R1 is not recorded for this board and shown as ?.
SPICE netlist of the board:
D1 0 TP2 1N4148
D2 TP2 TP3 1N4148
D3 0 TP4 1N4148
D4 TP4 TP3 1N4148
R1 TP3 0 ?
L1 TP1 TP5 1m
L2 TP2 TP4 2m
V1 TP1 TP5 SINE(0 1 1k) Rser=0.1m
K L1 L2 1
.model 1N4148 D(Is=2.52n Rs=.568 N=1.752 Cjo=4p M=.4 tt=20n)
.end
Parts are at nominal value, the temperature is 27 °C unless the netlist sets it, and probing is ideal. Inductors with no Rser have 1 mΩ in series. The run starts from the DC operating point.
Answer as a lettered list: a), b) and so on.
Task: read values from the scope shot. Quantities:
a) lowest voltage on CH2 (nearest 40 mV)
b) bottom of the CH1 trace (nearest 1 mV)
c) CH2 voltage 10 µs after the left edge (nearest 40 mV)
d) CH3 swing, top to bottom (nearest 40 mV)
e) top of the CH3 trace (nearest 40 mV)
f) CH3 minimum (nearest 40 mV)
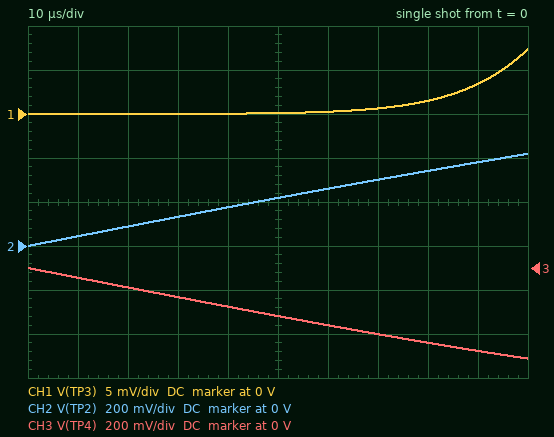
a) 0 V
b) 0 V
c) 40 mV
d) 400 mV
e) 0 V
f) -400 mV
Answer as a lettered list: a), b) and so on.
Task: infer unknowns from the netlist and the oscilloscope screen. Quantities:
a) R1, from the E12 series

a) 330 Ω
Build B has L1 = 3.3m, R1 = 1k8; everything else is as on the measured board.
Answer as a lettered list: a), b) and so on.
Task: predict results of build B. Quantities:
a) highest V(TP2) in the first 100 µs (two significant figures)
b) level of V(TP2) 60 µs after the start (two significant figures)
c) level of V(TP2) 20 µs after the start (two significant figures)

a) 230 mV
b) 140 mV
c) 49 mV
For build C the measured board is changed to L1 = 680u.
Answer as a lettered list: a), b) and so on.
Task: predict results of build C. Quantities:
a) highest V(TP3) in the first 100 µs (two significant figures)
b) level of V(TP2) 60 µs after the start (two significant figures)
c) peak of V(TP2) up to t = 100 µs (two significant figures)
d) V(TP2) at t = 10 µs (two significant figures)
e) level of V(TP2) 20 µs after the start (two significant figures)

a) 37 mV
b) 320 mV
c) 520 mV
d) 54 mV
e) 110 mV
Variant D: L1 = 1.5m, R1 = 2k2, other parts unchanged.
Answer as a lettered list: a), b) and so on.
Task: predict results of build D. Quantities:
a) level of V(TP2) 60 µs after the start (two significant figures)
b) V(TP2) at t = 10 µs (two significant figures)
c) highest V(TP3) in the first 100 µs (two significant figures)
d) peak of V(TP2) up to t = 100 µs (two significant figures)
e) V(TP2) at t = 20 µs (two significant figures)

a) 210 mV
b) 36 mV
c) 9.0 mV
d) 340 mV
e) 72 mV
